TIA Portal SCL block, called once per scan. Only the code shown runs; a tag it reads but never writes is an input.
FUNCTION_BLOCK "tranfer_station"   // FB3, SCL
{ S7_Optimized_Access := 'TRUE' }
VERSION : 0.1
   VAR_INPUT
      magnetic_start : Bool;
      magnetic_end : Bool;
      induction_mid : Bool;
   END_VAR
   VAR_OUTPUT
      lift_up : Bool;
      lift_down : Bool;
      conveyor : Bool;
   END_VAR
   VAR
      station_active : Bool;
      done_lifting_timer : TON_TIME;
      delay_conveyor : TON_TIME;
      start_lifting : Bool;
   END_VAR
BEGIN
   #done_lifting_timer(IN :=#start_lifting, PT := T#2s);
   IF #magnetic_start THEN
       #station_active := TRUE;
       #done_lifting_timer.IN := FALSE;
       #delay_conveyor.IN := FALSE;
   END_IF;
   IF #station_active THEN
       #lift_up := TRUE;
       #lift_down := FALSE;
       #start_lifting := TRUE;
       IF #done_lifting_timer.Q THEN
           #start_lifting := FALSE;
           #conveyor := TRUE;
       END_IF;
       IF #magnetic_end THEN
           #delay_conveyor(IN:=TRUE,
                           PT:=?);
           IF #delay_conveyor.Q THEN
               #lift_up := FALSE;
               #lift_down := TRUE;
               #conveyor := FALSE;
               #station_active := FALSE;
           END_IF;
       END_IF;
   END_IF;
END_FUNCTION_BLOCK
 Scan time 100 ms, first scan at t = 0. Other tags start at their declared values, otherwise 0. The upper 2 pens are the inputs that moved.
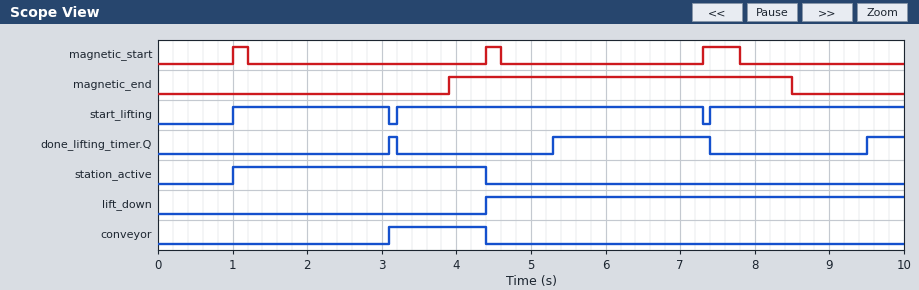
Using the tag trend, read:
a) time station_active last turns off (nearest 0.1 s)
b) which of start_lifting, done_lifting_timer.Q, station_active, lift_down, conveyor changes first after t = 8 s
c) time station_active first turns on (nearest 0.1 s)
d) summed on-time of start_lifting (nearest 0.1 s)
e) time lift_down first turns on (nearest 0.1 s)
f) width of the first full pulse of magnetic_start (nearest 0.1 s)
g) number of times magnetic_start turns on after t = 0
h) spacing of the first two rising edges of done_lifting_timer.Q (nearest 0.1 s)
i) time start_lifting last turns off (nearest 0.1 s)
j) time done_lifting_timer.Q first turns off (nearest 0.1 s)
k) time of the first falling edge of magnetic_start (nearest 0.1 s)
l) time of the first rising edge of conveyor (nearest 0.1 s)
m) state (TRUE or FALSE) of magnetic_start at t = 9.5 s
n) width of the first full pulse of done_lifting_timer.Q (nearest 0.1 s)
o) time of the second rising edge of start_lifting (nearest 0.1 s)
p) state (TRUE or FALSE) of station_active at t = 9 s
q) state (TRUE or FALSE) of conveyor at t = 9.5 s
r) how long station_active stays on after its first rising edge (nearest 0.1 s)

4.4 s
done_lifting_timer.Q
1.0 s
8.8 s
4.4 s
0.2 s
3
2.2 s
7.3 s
3.2 s
1.2 s
3.1 s
FALSE
0.1 s
3.2 s
FALSE
FALSE
3.4 s
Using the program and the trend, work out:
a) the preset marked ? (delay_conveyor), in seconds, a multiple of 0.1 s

0.5 s
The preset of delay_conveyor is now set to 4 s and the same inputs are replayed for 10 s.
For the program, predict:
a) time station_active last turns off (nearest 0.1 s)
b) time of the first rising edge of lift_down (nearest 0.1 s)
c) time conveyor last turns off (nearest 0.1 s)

7.9 s
7.9 s
7.9 s
